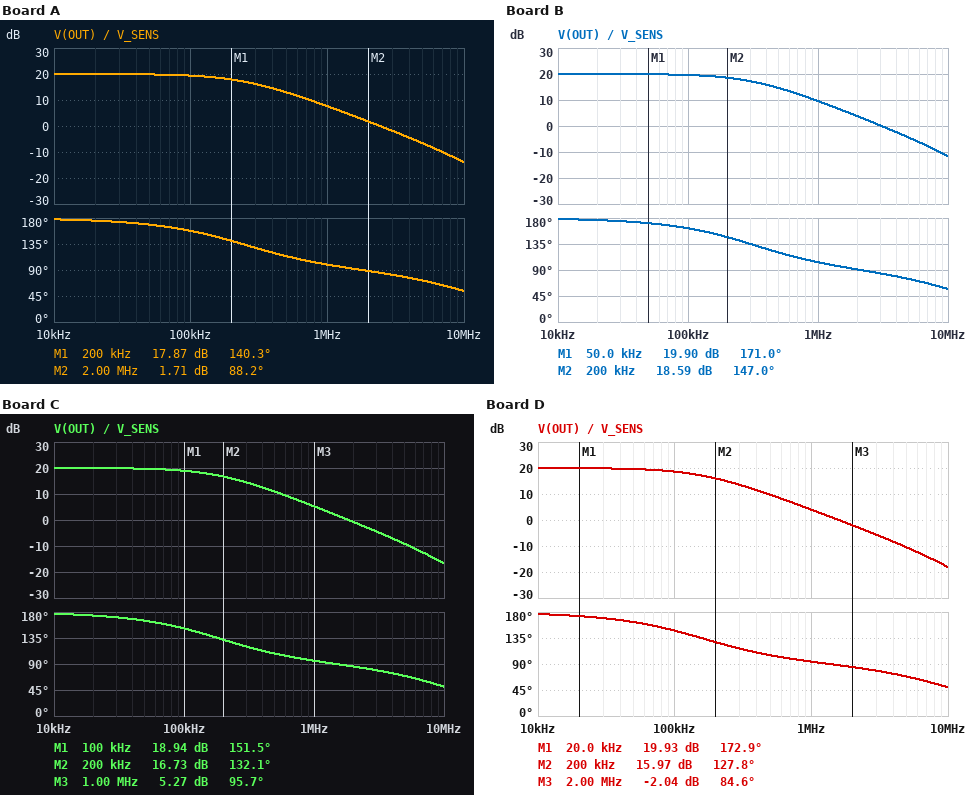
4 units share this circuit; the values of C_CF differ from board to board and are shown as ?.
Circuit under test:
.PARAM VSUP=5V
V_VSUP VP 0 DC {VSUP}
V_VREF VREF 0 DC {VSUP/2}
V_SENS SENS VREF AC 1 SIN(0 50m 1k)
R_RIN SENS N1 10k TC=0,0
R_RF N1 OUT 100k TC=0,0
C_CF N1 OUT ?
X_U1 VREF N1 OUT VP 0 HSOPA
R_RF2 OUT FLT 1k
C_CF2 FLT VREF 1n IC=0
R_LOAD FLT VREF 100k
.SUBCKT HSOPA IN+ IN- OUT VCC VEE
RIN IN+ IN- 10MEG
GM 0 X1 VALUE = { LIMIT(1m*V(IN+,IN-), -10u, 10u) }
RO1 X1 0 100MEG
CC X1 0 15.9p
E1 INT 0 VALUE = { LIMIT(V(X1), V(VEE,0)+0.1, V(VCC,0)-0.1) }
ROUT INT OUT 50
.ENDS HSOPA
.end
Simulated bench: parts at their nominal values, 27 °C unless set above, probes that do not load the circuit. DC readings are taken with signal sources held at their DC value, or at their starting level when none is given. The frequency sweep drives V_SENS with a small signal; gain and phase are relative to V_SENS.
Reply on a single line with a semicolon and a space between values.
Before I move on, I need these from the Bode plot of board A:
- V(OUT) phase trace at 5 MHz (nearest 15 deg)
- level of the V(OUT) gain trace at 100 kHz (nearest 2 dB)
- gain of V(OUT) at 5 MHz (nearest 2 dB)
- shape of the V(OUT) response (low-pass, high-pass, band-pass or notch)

75 deg; 20 dB; -6 dB; low-pass
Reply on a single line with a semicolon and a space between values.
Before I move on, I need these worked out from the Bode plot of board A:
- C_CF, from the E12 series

4.7 pF
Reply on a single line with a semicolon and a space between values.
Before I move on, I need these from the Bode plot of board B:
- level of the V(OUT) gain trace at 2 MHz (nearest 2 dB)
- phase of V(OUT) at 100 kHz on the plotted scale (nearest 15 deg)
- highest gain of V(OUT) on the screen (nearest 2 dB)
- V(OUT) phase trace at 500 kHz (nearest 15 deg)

4 dB; 165 deg; 20 dB; 120 deg
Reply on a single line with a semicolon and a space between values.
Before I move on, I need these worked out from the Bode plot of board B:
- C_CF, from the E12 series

3.3 pF
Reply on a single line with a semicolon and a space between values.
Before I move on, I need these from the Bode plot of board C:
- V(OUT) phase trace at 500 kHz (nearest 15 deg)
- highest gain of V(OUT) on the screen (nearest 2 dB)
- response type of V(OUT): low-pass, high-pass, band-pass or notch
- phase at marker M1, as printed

105 deg; 20 dB; low-pass; 151.5 deg
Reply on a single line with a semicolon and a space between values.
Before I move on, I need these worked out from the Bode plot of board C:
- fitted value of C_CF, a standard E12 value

6.8 pF
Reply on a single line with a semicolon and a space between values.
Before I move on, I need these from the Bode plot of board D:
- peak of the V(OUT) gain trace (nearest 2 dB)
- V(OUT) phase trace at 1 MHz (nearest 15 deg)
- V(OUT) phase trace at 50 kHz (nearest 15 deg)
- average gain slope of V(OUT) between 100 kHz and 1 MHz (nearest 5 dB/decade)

20 dB; 90 deg; 165 deg; -15 dB/decade
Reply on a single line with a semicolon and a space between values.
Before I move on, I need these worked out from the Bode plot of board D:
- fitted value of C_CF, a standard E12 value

8.2 pF
